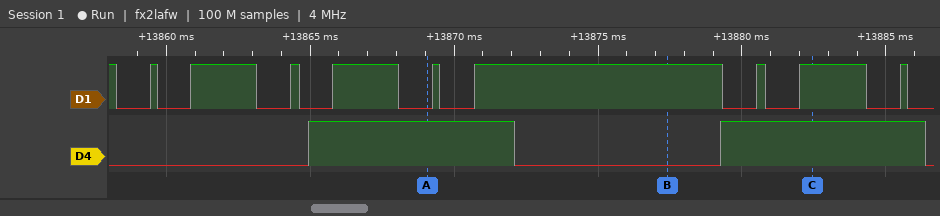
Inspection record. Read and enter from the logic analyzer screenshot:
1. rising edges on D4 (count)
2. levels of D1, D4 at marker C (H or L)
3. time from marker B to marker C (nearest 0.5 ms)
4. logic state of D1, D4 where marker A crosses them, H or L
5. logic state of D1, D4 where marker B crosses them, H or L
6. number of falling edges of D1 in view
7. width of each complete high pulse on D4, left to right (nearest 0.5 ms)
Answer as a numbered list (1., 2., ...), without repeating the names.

1. 2
2. D1=H, D4=H
3. 5 ms
4. D1=L, D4=H
5. D1=H, D4=L
6. 10
7. 7 ms, 7 ms
